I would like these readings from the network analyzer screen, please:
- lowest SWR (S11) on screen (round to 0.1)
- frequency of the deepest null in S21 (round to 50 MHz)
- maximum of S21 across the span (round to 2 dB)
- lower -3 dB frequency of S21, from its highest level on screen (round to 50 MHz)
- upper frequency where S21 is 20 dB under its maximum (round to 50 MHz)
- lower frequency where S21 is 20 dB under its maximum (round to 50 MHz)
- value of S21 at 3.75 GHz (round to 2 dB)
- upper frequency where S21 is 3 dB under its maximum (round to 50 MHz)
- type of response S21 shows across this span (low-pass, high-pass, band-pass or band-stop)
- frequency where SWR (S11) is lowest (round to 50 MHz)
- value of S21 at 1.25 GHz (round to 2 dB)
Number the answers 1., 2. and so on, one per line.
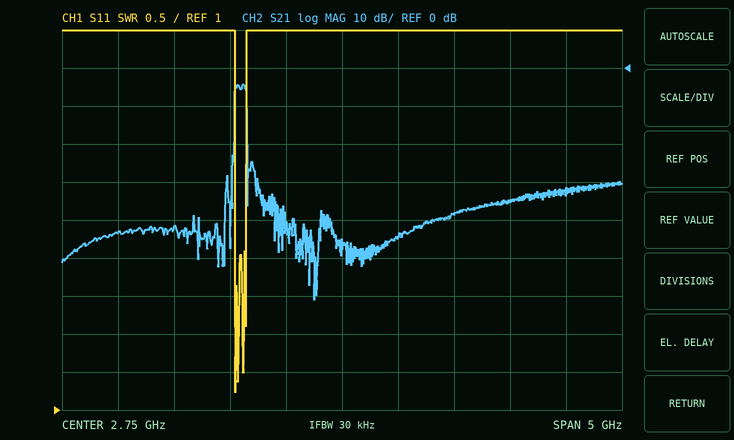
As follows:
1. 1.2
2. 2.50 GHz
3. -4 dB
4. 1.80 GHz
5. 1.90 GHz
6. 1.80 GHz
7. -38 dB
8. 1.90 GHz
9. band-pass
10. 1.80 GHz
11. -42 dB
